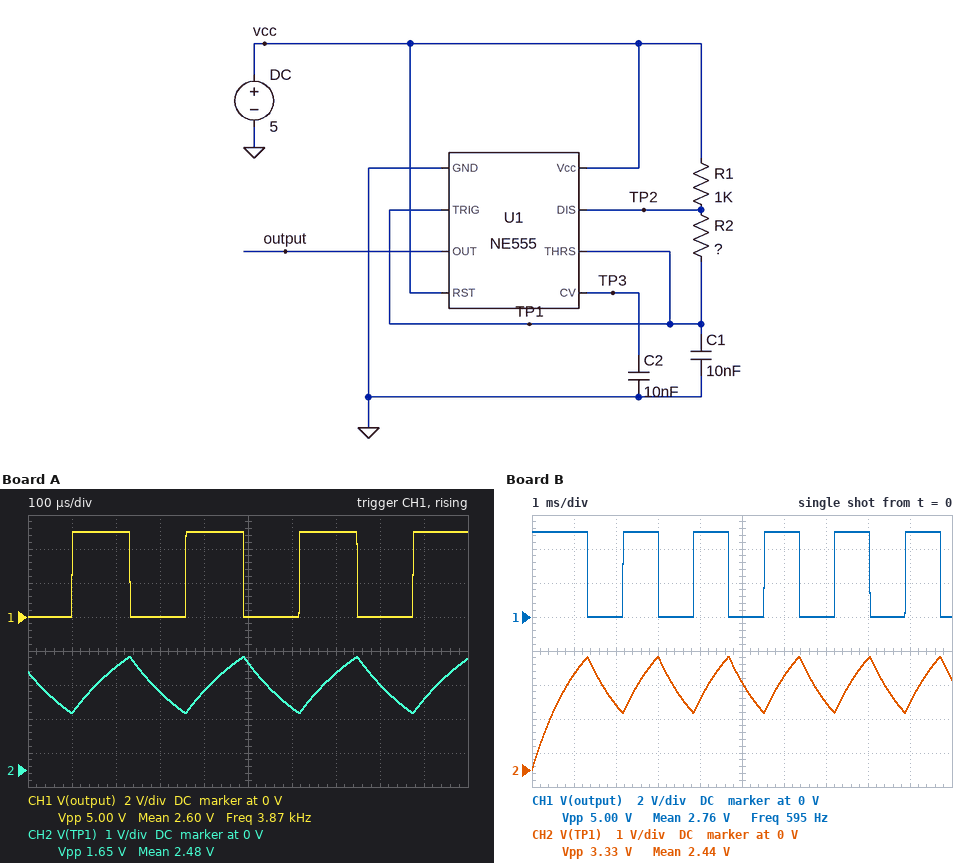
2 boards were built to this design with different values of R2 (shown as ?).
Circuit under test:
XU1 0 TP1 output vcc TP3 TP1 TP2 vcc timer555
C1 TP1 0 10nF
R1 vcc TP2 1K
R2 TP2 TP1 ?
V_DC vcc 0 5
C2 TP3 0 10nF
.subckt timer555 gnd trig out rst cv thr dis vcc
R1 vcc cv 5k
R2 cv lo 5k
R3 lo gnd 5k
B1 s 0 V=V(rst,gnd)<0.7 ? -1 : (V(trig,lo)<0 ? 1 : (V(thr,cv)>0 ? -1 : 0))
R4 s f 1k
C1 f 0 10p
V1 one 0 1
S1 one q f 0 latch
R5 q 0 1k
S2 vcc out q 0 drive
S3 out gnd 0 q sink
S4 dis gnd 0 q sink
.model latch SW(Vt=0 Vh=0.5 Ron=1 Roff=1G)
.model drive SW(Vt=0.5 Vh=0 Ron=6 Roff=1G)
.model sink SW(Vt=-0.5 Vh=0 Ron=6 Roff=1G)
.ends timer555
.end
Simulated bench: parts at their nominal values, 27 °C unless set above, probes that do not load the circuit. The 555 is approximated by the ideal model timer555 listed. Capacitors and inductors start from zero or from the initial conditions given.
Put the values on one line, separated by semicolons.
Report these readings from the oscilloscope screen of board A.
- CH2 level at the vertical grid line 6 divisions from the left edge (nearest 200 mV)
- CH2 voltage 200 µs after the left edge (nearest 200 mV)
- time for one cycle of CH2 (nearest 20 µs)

1.8 V; 3.0 V; 260 µs
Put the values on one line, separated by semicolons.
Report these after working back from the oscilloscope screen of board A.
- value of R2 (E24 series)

18 kΩ
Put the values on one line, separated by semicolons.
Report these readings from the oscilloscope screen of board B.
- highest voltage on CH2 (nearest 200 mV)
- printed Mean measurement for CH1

3.4 V; 2.76 V
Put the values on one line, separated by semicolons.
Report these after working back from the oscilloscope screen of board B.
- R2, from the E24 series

120 kΩ
